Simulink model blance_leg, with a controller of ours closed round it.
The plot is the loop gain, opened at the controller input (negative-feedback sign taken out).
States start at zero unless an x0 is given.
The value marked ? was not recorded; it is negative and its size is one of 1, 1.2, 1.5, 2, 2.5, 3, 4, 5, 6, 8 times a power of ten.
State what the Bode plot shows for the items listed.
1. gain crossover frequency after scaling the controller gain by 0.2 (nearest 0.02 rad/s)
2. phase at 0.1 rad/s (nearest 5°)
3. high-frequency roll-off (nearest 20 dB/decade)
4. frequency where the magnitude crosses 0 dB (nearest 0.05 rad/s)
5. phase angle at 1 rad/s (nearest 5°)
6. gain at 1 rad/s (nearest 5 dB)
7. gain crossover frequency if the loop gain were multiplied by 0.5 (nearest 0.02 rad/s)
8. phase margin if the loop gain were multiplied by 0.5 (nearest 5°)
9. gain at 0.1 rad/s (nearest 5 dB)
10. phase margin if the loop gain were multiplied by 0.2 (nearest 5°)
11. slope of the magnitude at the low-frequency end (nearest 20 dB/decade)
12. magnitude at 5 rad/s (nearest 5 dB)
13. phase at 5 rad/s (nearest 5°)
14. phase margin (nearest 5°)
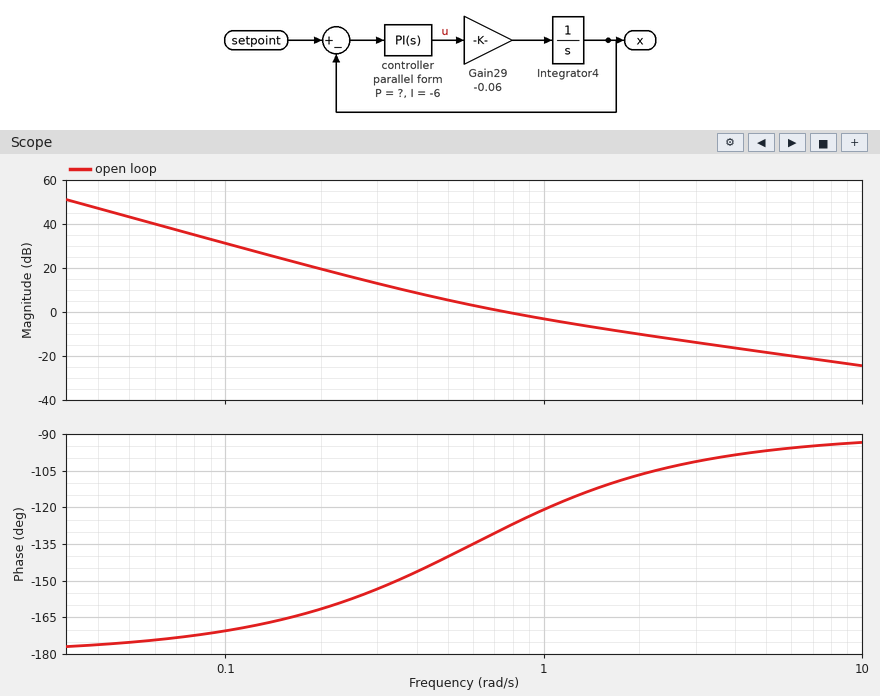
0.28 rad/s
-170°
-20 dB/decade
0.75 rad/s
-120°
-5 dB
0.48 rad/s
40°
30 dB
25°
-40 dB/decade
-20 dB
-95°
50°
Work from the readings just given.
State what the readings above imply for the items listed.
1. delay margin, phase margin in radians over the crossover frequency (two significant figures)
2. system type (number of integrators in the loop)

1.2 s
2
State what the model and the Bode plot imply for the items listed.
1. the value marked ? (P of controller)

-10
